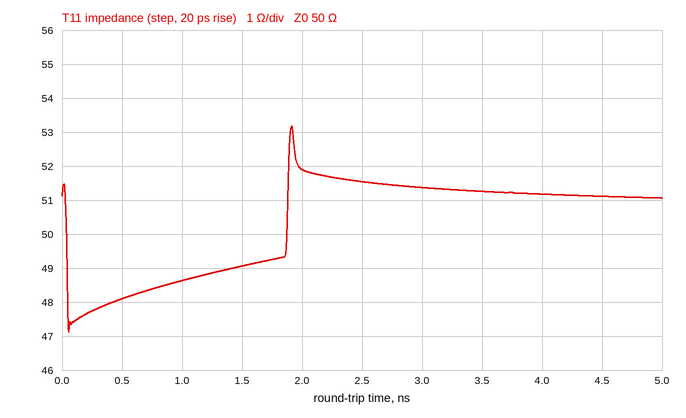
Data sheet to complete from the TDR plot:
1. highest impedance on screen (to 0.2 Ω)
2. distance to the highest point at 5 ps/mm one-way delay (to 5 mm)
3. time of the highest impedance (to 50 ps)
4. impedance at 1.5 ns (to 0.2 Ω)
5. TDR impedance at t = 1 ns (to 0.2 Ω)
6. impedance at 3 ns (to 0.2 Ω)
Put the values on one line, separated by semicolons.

53.2 Ω; 190 mm; 1.90 ns; 49.0 Ω; 48.6 Ω; 51.4 Ω
